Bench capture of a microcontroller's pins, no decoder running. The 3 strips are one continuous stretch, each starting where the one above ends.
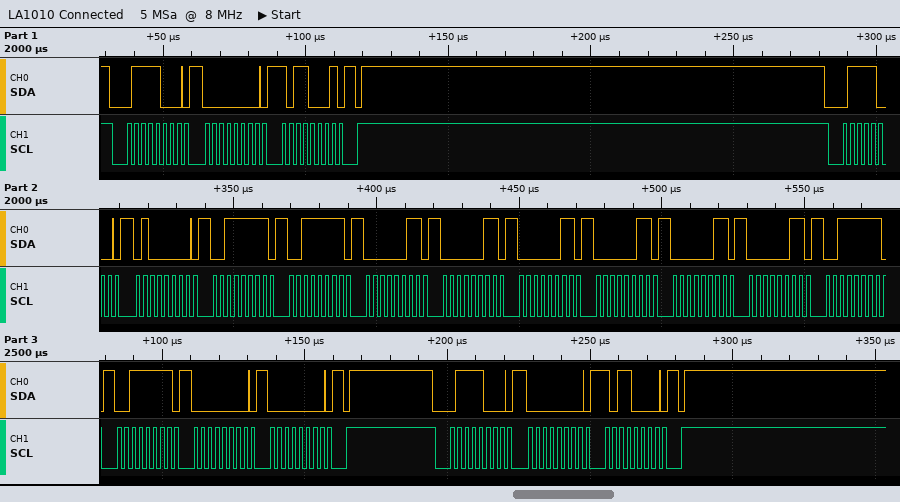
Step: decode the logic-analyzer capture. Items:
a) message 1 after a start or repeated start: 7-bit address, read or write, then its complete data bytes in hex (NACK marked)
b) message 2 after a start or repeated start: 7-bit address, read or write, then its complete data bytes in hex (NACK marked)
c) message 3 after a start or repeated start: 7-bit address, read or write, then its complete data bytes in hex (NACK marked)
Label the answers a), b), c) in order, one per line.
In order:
a) 0x3C write: 00 B1
b) 0x3C write: 40 3F 3F 03 03 03 03 03 03 3F 3F 00 00
c) 0x3C write: 00 B0
